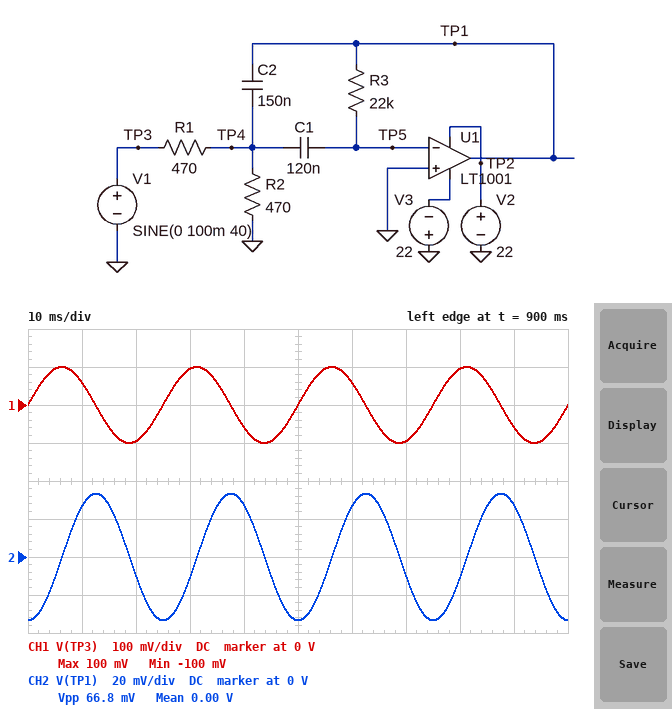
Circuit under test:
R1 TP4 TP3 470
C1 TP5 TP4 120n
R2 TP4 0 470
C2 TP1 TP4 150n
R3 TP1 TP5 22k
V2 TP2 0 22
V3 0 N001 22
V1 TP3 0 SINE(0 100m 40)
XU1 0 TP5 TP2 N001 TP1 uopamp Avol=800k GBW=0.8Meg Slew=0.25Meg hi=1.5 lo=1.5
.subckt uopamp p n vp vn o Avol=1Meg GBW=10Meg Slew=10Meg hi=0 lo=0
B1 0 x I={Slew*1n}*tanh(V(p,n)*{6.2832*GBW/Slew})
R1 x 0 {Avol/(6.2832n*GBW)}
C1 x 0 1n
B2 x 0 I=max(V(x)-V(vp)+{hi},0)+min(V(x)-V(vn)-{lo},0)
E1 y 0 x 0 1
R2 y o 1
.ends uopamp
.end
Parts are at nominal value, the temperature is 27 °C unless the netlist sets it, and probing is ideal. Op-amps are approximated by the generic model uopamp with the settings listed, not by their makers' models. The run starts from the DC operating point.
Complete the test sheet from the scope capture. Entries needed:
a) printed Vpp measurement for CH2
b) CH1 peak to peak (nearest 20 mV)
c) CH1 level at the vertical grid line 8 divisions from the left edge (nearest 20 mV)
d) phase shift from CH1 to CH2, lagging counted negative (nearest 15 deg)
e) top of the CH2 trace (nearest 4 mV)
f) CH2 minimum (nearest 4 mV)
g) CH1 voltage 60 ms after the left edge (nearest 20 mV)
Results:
66.8 mV
200 mV
100 mV
-90 deg
32 mV
-32 mV
60 mV
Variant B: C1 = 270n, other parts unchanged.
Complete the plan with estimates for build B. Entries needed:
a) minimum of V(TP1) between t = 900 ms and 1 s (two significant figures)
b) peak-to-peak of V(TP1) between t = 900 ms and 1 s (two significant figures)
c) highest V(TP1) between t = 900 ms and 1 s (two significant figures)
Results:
-76 mV
150 mV
76 mV
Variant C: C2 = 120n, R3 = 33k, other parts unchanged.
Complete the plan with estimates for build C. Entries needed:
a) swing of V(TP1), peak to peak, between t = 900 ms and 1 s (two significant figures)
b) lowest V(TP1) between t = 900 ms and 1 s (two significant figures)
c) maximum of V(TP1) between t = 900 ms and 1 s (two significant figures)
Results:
100 mV
-50 mV
50 mV
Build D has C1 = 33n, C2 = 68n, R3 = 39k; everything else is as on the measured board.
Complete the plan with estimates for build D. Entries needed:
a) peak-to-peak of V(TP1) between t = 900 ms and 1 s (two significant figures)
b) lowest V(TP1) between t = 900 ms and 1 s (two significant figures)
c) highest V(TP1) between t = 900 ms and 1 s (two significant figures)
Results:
32 mV
-16 mV
16 mV
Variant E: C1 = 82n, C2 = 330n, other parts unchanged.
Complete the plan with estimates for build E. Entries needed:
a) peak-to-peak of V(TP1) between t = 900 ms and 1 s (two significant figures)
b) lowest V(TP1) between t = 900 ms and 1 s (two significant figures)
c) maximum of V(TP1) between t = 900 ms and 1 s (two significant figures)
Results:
46 mV
-23 mV
23 mV
